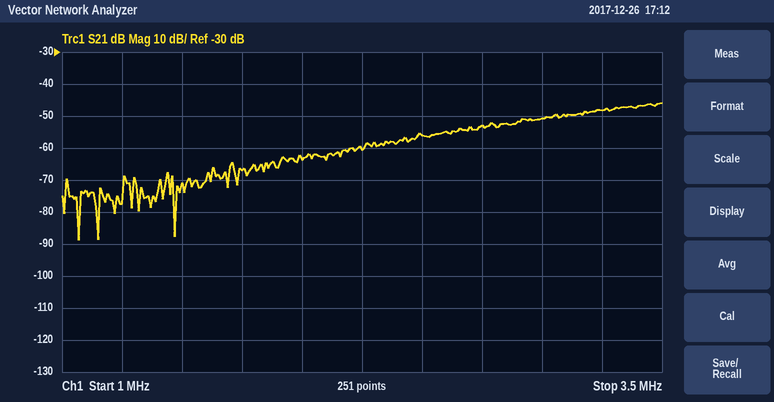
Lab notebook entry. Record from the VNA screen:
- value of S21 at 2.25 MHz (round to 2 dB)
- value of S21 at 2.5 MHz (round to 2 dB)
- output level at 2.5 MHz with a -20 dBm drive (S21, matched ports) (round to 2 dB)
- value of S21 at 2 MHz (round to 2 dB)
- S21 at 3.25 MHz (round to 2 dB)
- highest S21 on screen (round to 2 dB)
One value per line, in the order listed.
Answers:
-60 dB
-56 dB
-76 dBm
-64 dB
-48 dB
-46 dB
